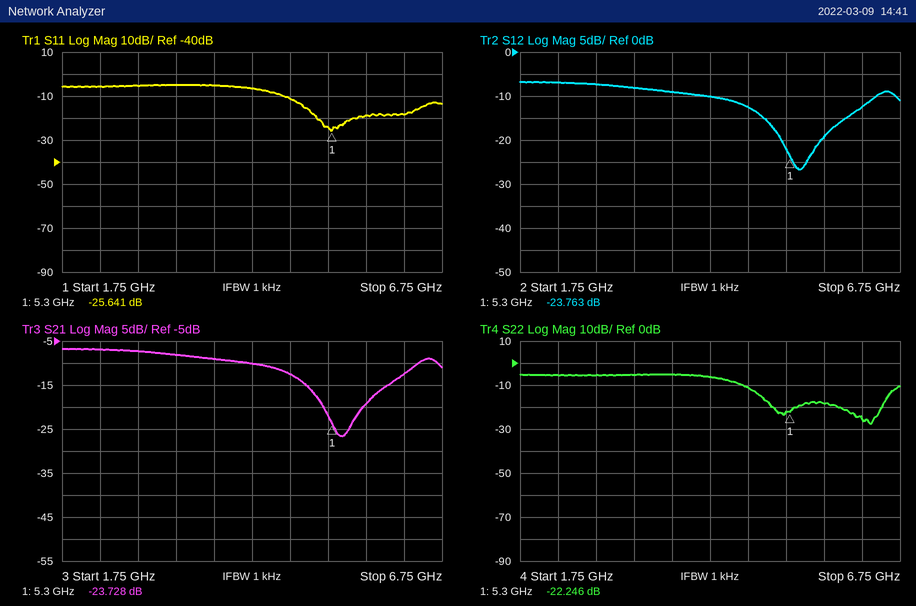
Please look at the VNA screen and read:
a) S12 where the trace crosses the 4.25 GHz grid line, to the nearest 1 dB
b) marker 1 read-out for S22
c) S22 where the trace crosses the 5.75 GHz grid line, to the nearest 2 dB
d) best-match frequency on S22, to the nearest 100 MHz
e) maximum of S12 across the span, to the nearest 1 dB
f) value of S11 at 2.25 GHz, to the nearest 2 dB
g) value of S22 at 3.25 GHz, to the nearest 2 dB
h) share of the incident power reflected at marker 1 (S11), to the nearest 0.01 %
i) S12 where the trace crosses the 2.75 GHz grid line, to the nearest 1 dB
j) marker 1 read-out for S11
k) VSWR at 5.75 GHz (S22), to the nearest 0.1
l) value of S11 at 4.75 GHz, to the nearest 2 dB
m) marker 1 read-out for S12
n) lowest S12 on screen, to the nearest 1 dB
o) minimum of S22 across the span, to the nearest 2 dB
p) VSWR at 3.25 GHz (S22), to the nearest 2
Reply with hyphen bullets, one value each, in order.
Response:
- -10 dB
- -22.246 dB
- -18 dB
- 6.4 GHz
- -7 dB
- -6 dB
- -6 dB
- 0.27 %
- -7 dB
- -25.641 dB
- 1.3
- -12 dB
- -23.763 dB
- -27 dB
- -28 dB
- 4
